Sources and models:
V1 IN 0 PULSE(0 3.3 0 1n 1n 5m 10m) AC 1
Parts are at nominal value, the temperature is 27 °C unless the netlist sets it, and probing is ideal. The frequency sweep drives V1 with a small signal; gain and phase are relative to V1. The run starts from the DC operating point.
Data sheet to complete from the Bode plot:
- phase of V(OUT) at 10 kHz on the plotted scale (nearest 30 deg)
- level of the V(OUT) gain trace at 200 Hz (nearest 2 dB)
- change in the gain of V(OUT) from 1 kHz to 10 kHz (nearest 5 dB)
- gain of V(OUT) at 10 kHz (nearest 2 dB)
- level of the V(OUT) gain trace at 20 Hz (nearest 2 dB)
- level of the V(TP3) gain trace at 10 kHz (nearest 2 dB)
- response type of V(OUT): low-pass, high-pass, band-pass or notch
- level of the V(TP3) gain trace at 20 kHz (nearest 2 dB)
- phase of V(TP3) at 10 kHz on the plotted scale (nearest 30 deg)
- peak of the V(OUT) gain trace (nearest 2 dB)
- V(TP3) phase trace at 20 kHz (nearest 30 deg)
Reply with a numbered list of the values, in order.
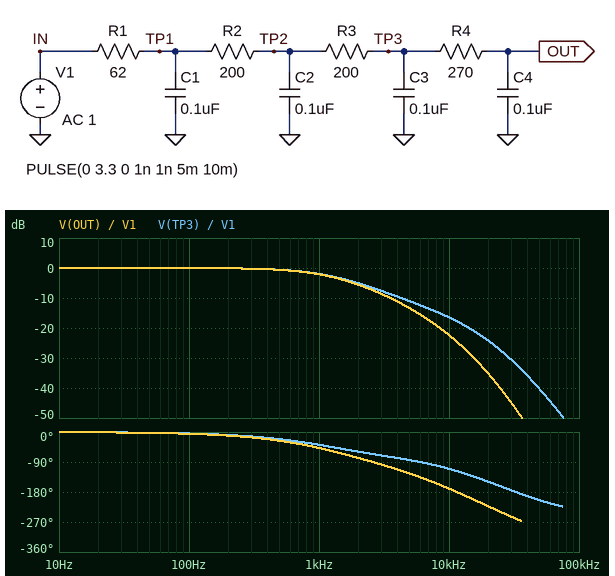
1. -180 deg
2. 0 dB
3. -20 dB
4. -22 dB
5. 0 dB
6. -16 dB
7. low-pass
8. -24 dB
9. -120 deg
10. 0 dB
11. -150 deg
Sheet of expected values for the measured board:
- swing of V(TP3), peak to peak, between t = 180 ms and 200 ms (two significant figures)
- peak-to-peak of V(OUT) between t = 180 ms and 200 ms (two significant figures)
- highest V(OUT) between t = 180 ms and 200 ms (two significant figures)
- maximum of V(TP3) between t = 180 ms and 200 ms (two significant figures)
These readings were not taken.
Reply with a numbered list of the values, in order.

1. 3.3 V
2. 3.3 V
3. 3.3 V
4. 3.3 V
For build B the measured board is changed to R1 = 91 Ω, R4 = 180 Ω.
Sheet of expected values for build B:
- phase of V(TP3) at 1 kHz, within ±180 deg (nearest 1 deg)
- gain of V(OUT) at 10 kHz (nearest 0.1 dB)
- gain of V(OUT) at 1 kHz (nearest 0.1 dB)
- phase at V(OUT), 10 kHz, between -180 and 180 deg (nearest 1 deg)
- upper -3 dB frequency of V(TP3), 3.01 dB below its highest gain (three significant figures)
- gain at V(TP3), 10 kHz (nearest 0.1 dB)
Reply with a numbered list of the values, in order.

1. -42 deg
2. -22.1 dB
3. -2.2 dB
4. -167 deg
5. 1.25 kHz
6. -18.5 dB
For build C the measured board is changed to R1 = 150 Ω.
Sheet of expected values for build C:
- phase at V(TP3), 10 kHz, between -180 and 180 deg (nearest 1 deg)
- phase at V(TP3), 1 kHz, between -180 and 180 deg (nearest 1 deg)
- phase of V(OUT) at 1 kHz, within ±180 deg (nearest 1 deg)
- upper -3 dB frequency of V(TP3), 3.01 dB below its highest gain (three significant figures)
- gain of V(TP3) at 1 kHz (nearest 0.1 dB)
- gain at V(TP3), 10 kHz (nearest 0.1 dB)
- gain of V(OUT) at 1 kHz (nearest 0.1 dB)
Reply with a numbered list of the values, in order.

1. -126 deg
2. -47 deg
3. -56 deg
4. 1.06 kHz
5. -2.8 dB
6. -19.8 dB
7. -2.9 dB
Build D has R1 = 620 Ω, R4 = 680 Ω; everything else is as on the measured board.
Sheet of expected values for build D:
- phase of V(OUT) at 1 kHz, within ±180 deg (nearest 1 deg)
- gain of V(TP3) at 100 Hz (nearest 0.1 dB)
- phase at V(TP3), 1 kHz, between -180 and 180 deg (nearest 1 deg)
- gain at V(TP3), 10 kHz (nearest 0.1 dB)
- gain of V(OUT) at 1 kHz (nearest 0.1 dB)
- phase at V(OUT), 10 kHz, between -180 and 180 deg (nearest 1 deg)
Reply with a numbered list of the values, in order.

1. -91 deg
2. -0.2 dB
3. -68 deg
4. -27.8 dB
5. -8.0 dB
6. 135 deg
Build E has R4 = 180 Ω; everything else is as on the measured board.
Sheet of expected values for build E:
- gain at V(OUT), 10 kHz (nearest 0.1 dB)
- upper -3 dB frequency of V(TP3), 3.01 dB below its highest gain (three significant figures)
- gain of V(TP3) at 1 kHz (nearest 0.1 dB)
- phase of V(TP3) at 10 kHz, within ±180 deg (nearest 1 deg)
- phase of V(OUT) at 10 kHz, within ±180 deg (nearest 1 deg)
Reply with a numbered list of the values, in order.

1. -20.9 dB
2. 1.35 kHz
3. -1.9 dB
4. -112 deg
5. -160 deg
